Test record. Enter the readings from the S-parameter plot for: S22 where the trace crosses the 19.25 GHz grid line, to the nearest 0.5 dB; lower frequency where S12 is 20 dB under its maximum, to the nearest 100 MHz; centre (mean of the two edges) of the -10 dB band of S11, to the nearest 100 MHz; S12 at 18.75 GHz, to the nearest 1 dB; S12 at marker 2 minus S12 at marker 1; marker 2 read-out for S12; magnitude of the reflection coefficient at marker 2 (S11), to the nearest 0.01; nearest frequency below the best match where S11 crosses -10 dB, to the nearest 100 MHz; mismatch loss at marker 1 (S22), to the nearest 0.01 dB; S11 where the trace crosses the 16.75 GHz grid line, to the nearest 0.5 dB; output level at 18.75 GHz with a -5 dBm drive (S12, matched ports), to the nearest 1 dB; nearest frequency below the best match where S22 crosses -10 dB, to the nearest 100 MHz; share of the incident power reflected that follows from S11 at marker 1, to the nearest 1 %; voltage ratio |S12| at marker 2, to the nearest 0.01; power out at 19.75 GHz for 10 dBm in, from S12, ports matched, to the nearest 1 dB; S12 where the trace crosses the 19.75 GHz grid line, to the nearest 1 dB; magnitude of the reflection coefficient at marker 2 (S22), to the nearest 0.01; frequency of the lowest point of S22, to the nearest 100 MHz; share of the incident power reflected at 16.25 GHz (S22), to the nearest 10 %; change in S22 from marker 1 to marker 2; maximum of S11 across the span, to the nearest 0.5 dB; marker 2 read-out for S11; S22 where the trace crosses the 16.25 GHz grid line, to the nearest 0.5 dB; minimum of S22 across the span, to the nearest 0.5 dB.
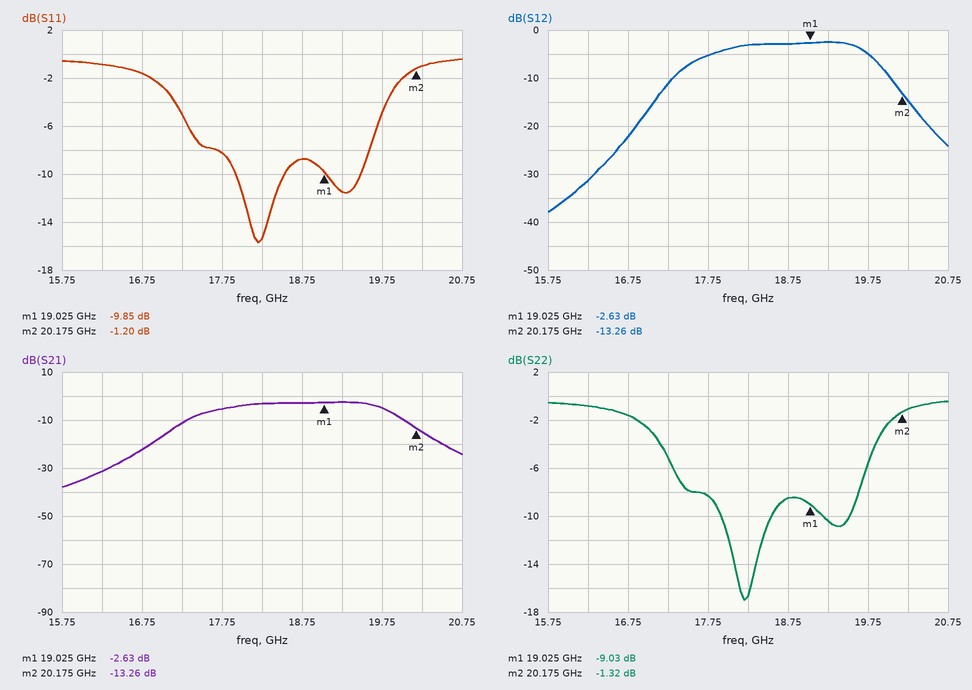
-10.5 dB
16.7 GHz
18.2 GHz
-3 dB
-10.63 dB
-13.26 dB
0.87
17.9 GHz
0.58 dB
-1.5 dB
-8 dBm
17.9 GHz
10 %
0.22
5 dBm
-5 dB
0.86
18.2 GHz
80 %
7.71 dB
-0.5 dB
-1.20 dB
-1.0 dB
-17.0 dB
